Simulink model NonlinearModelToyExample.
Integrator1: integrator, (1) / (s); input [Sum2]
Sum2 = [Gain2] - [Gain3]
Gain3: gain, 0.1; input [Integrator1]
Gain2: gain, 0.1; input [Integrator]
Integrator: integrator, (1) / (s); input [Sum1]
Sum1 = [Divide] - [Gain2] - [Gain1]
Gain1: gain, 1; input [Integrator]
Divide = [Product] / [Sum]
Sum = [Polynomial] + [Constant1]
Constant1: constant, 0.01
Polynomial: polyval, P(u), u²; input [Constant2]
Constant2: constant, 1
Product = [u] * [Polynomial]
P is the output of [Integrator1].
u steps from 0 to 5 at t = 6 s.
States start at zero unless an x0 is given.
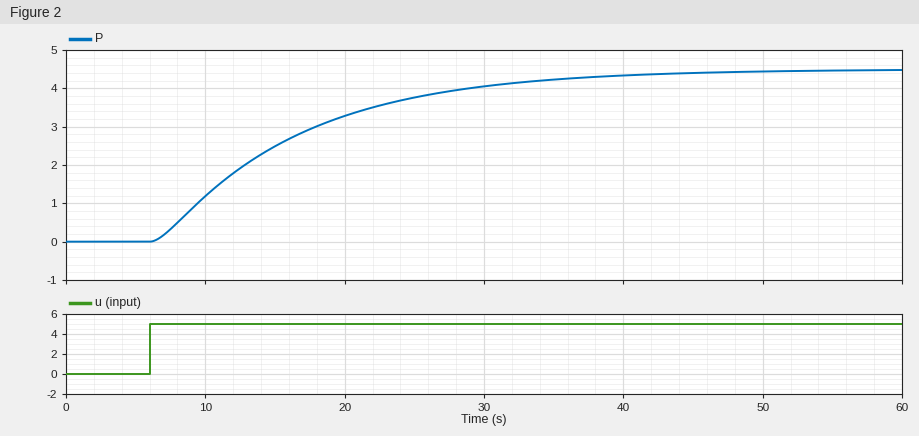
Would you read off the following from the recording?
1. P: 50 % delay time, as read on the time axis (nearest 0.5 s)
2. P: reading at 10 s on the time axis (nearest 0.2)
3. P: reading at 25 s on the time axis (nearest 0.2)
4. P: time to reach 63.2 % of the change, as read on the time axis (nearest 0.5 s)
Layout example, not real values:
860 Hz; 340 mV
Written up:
14.0 s; 1.2; 3.8; 17.0 s
